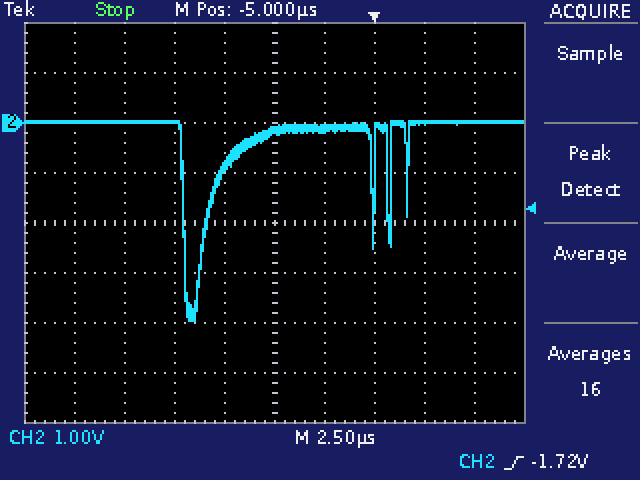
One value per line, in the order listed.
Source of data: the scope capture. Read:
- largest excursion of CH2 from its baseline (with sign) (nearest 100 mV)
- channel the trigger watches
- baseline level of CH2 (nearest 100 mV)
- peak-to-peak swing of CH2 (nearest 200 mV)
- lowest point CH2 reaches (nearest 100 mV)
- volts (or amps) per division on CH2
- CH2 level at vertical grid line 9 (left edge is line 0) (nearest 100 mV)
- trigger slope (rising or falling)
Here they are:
-4.0 V
CH2
0.0 V
4.0 V
-4.0 V
1 V
0.0 V
rising
